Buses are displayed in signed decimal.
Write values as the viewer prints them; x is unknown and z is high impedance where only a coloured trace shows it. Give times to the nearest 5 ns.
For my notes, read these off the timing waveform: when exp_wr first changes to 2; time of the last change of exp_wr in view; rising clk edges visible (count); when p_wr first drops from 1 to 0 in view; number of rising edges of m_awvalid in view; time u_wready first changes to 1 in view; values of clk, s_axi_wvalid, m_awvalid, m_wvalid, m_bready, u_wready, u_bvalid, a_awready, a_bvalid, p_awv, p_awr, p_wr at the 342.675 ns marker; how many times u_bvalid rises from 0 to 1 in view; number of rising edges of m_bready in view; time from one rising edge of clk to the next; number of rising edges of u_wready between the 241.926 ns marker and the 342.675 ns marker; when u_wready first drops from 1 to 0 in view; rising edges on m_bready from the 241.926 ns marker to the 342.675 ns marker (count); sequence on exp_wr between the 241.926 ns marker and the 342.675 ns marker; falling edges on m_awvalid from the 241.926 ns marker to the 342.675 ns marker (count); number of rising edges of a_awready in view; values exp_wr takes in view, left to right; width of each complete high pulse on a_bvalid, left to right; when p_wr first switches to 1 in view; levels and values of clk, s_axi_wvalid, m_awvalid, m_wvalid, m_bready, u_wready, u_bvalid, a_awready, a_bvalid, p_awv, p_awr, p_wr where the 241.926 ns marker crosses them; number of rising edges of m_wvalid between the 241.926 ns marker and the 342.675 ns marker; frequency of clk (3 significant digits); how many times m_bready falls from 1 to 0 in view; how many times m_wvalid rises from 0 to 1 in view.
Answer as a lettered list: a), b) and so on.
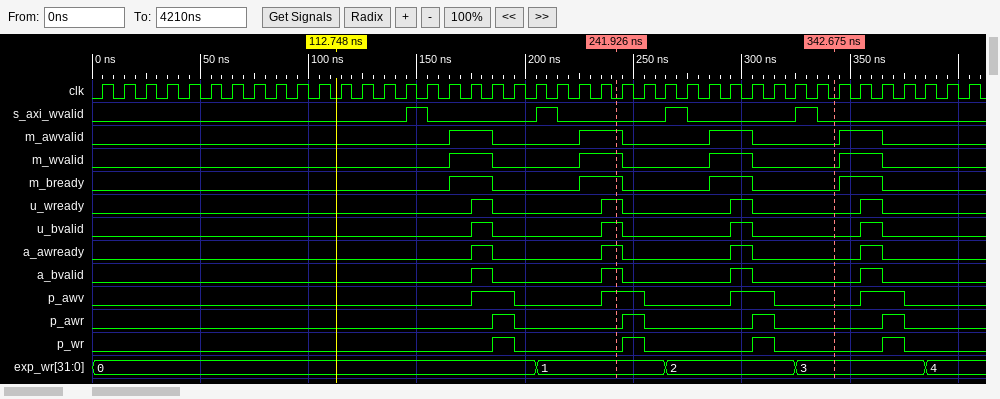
a) 265 ns
b) 385 ns
c) 41
d) 195 ns
e) 4
f) 175 ns
g) clk=0, s_axi_wvalid=0, m_awvalid=0, m_wvalid=0, m_bready=0, u_wready=0, u_bvalid=0, a_awready=0, a_bvalid=0, p_awv=0, p_awr=0, p_wr=0
h) 4
i) 4
j) 10 ns
k) 1
l) 185 ns
m) 1
n) 1, 2, 3
o) 2
p) 4
q) 0, 1, 2, 3, 4
r) 10 ns, 10 ns, 10 ns, 10 ns
s) 185 ns
t) clk=0, s_axi_wvalid=0, m_awvalid=1, m_wvalid=1, m_bready=1, u_wready=1, u_bvalid=1, a_awready=1, a_bvalid=1, p_awv=1, p_awr=0, p_wr=0
u) 1
v) 100 MHz
w) 4
x) 4
